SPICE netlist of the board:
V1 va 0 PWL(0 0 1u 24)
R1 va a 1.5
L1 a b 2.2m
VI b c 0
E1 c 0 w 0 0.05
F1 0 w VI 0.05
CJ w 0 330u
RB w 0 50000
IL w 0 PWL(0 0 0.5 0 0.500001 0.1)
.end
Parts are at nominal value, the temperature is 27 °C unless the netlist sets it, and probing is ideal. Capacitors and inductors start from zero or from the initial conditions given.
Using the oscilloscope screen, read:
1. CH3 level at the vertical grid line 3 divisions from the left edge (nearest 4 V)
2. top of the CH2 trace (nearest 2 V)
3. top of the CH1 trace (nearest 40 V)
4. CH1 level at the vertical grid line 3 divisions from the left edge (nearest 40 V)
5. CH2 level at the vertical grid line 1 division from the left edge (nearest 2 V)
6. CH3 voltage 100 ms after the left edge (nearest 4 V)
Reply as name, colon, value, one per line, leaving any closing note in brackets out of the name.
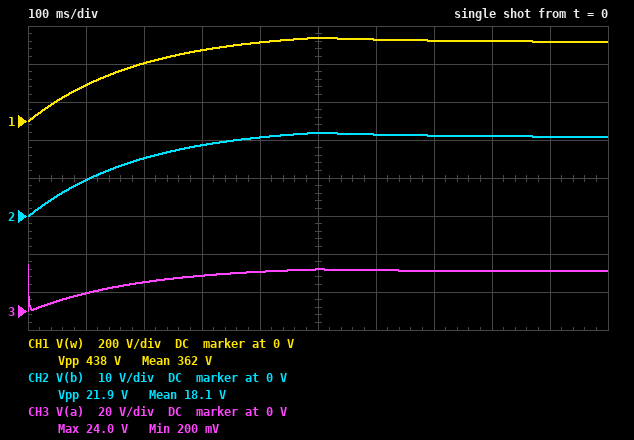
CH3 level at the vertical grid line 3 divisions from the left edge: 20 V
top of the CH2 trace: 22 V
top of the CH1 trace: 440 V
CH1 level at the vertical grid line 3 divisions from the left edge: 360 V
CH2 level at the vertical grid line 1 division from the left edge: 10 V
CH3 voltage 100 ms after the left edge: 8 V
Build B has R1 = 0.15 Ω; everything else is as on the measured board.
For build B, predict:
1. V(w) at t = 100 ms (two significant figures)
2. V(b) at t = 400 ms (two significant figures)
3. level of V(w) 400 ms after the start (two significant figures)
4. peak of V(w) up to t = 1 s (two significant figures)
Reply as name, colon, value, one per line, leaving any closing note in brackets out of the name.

V(w) at t = 100 ms: 490 V
V(b) at t = 400 ms: 24 V
level of V(w) 400 ms after the start: 480 V
peak of V(w) up to t = 1 s: 530 V
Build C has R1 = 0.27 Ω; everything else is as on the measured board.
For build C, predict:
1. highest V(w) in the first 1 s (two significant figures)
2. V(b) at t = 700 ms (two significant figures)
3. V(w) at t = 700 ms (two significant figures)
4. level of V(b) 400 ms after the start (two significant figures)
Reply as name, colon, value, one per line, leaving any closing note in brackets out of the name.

highest V(w) in the first 1 s: 480 V
V(b) at t = 700 ms: 23 V
V(w) at t = 700 ms: 470 V
level of V(b) 400 ms after the start: 24 V
